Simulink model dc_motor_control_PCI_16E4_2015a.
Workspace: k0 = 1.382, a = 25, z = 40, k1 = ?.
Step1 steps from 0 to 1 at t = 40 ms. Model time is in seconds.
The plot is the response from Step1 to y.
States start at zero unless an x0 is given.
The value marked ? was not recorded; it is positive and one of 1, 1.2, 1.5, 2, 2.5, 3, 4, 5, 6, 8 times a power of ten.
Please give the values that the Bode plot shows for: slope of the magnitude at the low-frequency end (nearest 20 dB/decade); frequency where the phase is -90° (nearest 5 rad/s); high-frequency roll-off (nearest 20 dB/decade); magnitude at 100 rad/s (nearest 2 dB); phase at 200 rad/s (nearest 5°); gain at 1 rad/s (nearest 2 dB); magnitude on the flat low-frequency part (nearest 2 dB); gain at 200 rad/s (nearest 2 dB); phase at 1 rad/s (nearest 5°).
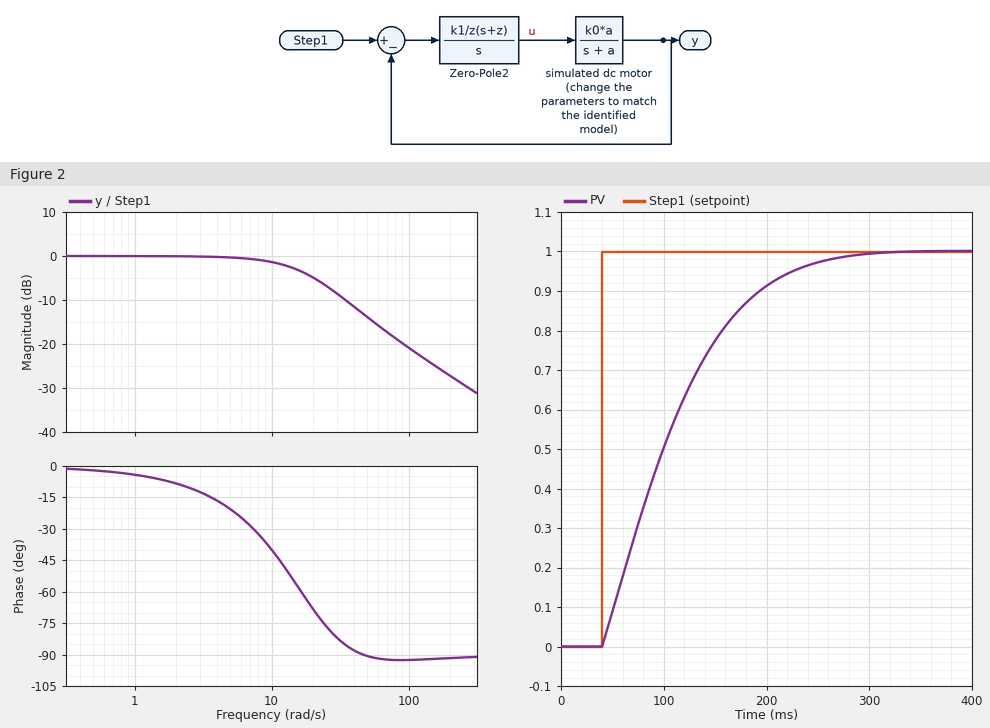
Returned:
0 dB/decade
45 rad/s
-20 dB/decade
-20 dB
-90°
0 dB
0 dB
-28 dB
-5°
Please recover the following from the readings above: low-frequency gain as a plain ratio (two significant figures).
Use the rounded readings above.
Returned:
1.0
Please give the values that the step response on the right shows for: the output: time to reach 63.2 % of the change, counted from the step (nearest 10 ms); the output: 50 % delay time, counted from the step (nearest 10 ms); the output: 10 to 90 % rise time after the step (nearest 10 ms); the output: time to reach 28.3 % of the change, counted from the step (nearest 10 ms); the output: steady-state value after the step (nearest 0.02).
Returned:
80 ms
60 ms
140 ms
30 ms
1.00
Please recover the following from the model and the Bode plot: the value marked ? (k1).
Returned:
10
